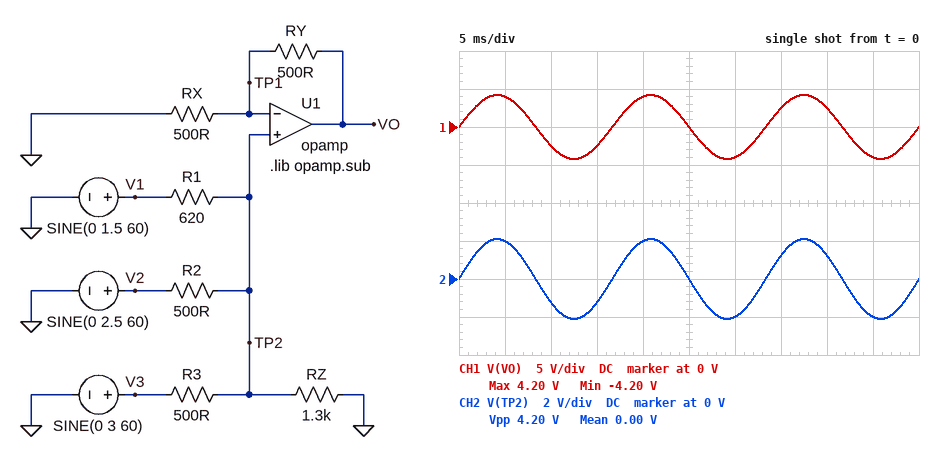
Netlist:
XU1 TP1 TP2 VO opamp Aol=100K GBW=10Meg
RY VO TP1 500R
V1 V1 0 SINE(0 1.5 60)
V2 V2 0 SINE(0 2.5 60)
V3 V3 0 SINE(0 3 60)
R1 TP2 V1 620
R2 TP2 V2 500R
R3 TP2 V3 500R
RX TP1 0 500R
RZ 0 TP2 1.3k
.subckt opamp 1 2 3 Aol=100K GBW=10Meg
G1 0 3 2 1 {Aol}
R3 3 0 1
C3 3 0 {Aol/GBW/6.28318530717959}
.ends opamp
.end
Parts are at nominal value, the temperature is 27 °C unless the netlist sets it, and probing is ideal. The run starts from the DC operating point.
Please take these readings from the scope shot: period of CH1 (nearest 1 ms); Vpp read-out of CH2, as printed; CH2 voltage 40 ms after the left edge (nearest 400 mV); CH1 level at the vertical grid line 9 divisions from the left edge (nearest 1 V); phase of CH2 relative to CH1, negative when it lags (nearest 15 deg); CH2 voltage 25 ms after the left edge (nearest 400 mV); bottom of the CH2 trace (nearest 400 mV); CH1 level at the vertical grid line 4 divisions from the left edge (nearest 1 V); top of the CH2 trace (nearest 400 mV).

17 ms
4.20 V
1.2 V
-4 V
0 deg
0 V
-2.0 V
4 V
2.0 V
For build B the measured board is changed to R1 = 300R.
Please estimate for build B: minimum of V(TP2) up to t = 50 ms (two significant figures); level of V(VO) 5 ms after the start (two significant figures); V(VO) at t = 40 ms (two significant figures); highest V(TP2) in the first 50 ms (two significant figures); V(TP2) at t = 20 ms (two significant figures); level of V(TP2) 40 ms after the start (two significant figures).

-2.0 V
3.8 V
2.3 V
2.0 V
1.9 V
1.2 V
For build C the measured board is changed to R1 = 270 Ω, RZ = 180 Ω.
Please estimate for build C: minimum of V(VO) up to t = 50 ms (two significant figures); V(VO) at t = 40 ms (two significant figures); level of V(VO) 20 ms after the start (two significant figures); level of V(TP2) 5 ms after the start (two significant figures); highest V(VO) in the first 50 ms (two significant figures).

-2.5 V
1.5 V
2.4 V
1.2 V
2.5 V
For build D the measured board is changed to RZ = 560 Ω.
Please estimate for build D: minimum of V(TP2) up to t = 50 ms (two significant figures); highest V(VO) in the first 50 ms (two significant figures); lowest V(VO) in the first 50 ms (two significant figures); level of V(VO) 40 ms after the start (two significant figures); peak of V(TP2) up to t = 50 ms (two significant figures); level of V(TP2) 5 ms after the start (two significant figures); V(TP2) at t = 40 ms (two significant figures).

-1.8 V
3.6 V
-3.6 V
2.1 V
1.8 V
1.7 V
1.1 V
